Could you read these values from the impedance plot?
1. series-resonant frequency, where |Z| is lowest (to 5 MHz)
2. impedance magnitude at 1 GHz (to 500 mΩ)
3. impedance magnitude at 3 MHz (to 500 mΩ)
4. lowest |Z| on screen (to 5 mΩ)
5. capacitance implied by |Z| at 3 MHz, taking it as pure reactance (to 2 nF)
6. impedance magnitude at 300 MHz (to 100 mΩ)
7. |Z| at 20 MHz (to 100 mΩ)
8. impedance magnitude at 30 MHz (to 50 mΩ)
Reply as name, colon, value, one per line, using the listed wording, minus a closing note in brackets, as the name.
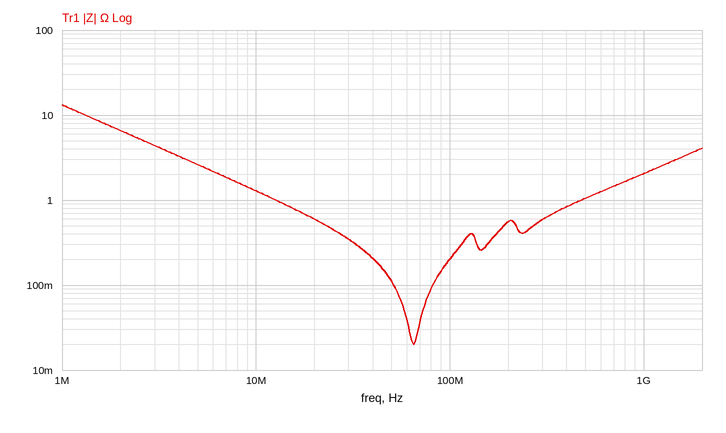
series-resonant frequency, where |Z| is lowest: 65 MHz
impedance magnitude at 1 GHz: 2.0 Ω
impedance magnitude at 3 MHz: 4.5 Ω
lowest |Z| on screen: 20 mΩ
capacitance implied by |Z| at 3 MHz, taking it as pure reactance: 12 nF
impedance magnitude at 300 MHz: 600 mΩ
|Z| at 20 MHz: 600 mΩ
impedance magnitude at 30 MHz: 350 mΩ
